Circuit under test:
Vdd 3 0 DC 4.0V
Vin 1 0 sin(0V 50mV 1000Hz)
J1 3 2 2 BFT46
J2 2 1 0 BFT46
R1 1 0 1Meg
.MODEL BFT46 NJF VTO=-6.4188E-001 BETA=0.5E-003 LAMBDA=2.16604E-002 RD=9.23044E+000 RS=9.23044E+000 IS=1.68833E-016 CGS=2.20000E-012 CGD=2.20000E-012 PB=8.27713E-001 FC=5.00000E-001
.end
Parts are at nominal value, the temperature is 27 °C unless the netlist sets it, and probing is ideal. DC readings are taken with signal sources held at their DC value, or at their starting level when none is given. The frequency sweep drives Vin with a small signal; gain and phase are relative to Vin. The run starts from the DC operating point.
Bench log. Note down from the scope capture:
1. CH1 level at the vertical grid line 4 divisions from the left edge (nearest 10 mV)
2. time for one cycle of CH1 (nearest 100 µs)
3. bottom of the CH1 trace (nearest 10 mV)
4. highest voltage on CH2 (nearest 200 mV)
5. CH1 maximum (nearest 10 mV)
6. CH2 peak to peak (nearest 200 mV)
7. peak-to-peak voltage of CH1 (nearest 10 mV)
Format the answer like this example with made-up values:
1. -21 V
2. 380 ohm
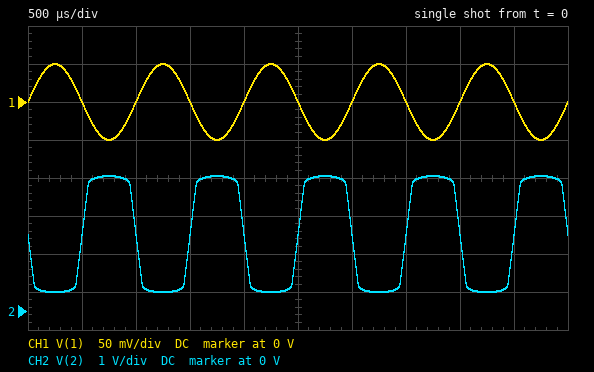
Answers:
1. 0 V
2. 1.0 ms
3. -50 mV
4. 3.6 V
5. 50 mV
6. 3.0 V
7. 100 mV
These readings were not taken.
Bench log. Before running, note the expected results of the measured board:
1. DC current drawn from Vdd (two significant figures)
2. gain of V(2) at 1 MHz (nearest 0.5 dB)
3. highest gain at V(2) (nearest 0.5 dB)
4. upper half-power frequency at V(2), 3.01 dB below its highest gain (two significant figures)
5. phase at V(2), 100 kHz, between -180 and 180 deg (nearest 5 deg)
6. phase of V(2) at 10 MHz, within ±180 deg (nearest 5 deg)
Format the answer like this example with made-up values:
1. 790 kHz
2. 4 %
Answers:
1. 210 µA
2. 31.5 dB
3. 37.5 dB
4. 590 kHz
5. 170 deg
6. 85 deg
